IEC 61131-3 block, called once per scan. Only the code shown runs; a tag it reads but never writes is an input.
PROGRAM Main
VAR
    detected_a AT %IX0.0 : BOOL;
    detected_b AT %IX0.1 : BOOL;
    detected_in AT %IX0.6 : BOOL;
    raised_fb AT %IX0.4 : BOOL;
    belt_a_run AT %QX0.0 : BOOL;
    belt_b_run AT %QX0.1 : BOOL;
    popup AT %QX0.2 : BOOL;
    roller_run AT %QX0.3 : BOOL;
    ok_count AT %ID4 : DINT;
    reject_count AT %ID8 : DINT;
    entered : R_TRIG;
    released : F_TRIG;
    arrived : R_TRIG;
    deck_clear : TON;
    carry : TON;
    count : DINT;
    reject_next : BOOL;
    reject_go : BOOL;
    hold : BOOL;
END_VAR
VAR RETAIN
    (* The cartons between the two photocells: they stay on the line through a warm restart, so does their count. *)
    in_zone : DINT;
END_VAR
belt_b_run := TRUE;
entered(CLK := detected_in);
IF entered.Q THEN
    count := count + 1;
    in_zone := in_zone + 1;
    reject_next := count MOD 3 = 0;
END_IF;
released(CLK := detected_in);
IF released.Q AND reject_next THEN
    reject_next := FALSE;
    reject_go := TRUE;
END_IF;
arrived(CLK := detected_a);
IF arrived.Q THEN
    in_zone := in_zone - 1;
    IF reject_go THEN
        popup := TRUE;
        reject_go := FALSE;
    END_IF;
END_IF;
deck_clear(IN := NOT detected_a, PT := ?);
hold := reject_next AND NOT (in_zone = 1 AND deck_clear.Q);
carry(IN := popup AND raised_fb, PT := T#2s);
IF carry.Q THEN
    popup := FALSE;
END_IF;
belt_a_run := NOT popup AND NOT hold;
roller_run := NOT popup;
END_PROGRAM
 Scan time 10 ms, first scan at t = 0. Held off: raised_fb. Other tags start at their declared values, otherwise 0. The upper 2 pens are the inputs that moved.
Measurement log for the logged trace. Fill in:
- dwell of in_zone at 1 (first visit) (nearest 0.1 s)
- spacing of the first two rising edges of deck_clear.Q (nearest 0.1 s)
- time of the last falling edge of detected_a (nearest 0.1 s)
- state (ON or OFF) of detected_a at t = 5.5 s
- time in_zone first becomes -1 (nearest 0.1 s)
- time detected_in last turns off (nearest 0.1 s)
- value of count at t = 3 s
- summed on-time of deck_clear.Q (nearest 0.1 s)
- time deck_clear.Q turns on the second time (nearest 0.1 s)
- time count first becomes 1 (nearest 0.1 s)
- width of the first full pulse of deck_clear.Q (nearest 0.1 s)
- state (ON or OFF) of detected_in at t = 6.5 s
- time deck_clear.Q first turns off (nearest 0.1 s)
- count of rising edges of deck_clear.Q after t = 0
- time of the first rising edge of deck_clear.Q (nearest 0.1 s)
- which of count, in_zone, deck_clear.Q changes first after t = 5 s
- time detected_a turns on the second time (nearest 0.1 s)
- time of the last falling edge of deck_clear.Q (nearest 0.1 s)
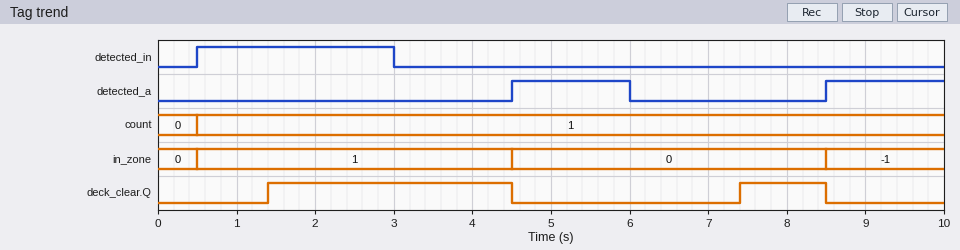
4.0 s
6.0 s
6.0 s
ON
8.5 s
3.0 s
1
4.2 s
7.4 s
0.5 s
3.1 s
OFF
4.5 s
2
1.4 s
deck_clear.Q
8.5 s
8.5 s
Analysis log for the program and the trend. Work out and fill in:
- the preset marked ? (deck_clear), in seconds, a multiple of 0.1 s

1.4 s
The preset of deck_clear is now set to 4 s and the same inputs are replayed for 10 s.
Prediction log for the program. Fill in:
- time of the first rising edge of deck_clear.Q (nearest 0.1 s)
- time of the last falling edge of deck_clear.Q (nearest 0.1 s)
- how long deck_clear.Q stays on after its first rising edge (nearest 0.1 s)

4.0 s
4.5 s
0.5 s
